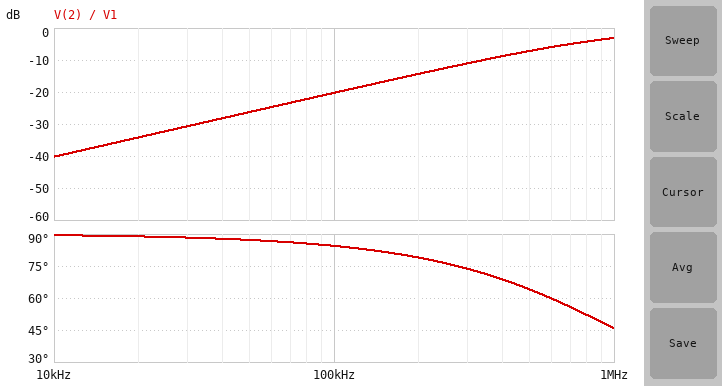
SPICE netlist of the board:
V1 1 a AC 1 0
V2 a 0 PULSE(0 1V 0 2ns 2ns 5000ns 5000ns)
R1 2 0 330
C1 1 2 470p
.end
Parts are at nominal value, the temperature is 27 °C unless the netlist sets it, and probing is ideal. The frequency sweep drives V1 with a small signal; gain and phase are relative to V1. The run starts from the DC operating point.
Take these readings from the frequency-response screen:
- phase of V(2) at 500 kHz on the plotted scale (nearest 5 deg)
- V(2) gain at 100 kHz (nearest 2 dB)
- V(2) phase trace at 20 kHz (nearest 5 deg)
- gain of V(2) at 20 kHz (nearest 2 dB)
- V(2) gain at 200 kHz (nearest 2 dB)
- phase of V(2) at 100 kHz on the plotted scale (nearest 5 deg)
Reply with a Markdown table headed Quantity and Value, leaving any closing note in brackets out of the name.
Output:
| Quantity | Value |
|---|---|
| phase of V(2) at 500 kHz on the plotted scale | 65 deg |
| V(2) gain at 100 kHz | -20 dB |
| V(2) phase trace at 20 kHz | 90 deg |
| gain of V(2) at 20 kHz | -34 dB |
| V(2) gain at 200 kHz | -14 dB |
| phase of V(2) at 100 kHz on the plotted scale | 85 deg |
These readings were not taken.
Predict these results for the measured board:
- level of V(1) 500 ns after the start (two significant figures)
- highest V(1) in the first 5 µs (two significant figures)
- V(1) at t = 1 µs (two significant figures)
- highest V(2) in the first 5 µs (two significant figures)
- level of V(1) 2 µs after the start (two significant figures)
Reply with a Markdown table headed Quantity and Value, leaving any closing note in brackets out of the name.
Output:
| Quantity | Value |
|---|---|
| level of V(1) 500 ns after the start | 1.0 V |
| highest V(1) in the first 5 µs | 1.0 V |
| V(1) at t = 1 µs | 1.0 V |
| highest V(2) in the first 5 µs | 990 mV |
| level of V(1) 2 µs after the start | 1.0 V |
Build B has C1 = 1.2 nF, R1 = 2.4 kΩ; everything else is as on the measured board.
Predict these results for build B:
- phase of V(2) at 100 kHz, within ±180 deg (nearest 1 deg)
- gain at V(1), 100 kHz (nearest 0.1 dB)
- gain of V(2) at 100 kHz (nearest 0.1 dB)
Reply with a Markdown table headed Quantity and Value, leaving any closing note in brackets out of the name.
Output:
| Quantity | Value |
|---|---|
| phase of V(2) at 100 kHz, within ±180 deg | 29 deg |
| gain at V(1), 100 kHz | 0 dB |
| gain of V(2) at 100 kHz | -1.2 dB |
